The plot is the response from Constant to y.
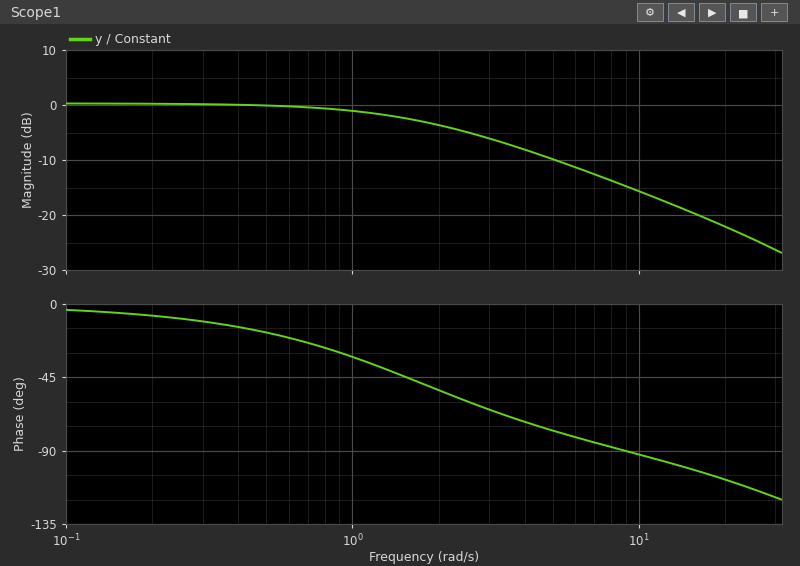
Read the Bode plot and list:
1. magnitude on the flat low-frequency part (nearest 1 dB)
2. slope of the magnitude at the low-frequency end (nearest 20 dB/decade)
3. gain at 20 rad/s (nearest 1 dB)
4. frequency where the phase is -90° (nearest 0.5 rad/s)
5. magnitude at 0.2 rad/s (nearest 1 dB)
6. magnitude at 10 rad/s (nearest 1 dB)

0 dB
0 dB/decade
-22 dB
9.0 rad/s
0 dB
-16 dB
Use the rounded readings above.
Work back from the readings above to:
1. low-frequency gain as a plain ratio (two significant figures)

1.0
